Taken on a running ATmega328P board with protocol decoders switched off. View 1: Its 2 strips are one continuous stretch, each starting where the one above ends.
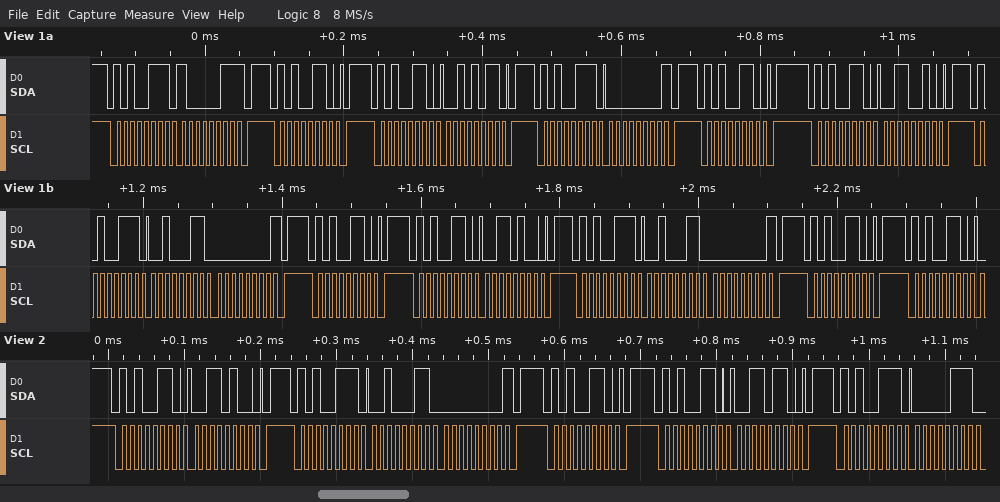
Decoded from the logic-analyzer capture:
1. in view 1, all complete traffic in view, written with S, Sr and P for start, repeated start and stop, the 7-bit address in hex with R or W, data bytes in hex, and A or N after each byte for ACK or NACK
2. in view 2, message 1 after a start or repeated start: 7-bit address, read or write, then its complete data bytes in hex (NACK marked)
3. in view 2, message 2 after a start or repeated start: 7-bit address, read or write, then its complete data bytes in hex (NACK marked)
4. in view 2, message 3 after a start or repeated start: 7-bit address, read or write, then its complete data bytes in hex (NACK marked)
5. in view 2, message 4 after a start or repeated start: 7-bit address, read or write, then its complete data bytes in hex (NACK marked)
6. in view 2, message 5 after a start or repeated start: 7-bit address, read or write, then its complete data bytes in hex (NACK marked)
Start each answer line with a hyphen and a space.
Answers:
- S 53R A 83 N P S 53W A P S 53W A 2B A P S 53R A 00 N P S 53W A P S 53W A 32 A P S 53R A 23 A 00 N P S 53W A P S 53W A 34 A P S 53R A 23 A 00 N P S 53W A P S 53W A
- 0x53 write: 34
- 0x53 read: 23 00 NACK
- 0x53 write
- 0x53 write: 36
- 0x53 read: 07
